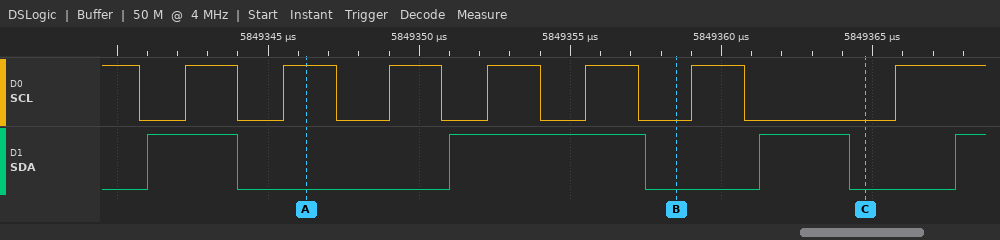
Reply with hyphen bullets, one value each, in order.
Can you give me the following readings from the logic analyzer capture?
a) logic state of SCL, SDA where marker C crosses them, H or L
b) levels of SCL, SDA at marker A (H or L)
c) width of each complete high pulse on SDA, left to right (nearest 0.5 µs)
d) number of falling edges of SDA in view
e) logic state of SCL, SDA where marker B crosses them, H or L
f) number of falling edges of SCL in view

- SCL=L, SDA=L
- SCL=H, SDA=L
- 3 µs, 6.5 µs, 3 µs
- 3
- SCL=L, SDA=L
- 7
